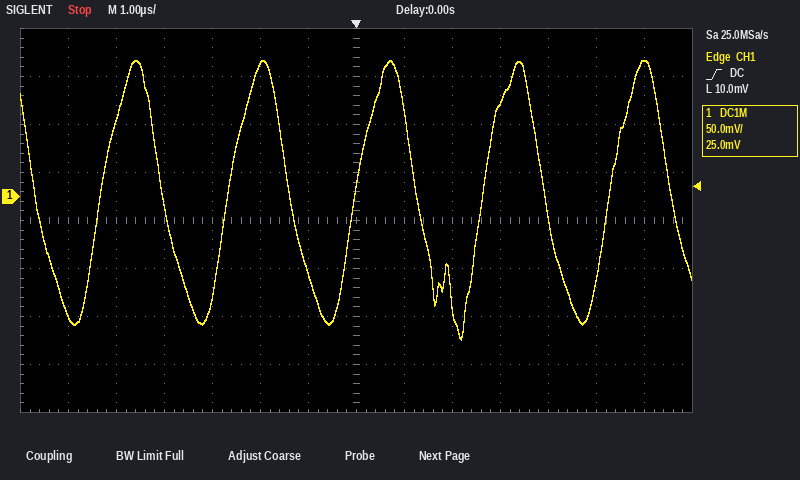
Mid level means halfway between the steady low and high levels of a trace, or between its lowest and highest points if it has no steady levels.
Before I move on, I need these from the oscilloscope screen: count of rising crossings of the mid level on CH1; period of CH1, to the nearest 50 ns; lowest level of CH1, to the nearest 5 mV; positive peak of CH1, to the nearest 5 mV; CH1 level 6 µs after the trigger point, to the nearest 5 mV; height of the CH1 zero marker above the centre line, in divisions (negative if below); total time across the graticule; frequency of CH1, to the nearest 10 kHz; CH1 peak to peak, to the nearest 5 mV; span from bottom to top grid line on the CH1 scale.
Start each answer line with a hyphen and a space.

- 5
- 2.65 µs
- -150 mV
- 140 mV
- 140 mV
- +0.5 div
- 14 µs
- 380 kHz
- 290 mV
- 400 mV
